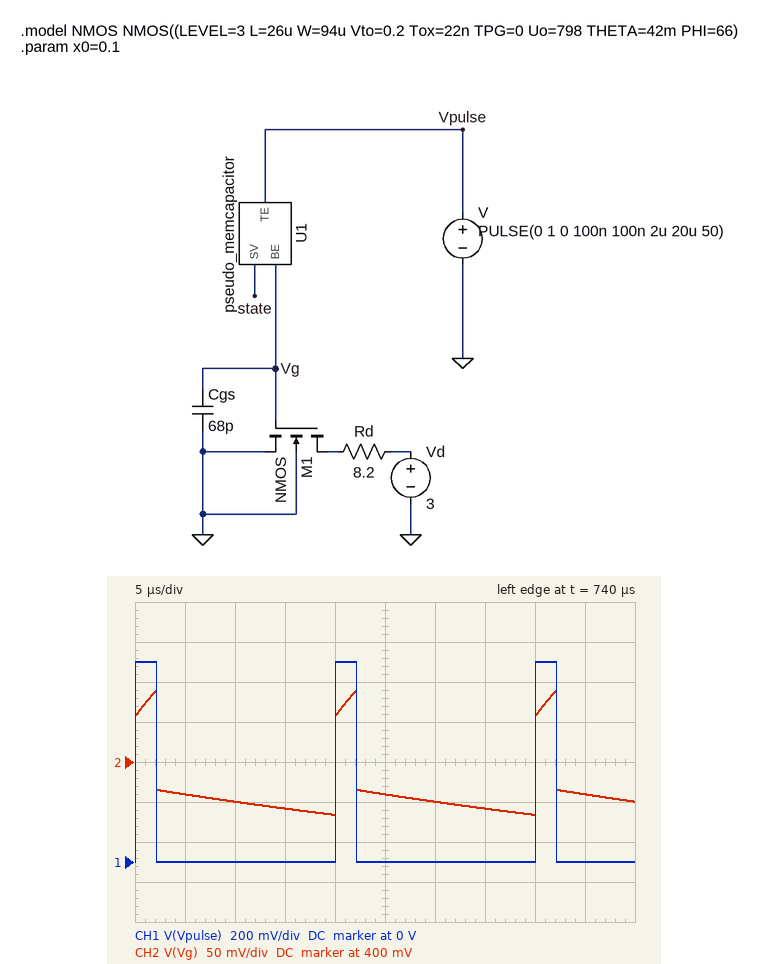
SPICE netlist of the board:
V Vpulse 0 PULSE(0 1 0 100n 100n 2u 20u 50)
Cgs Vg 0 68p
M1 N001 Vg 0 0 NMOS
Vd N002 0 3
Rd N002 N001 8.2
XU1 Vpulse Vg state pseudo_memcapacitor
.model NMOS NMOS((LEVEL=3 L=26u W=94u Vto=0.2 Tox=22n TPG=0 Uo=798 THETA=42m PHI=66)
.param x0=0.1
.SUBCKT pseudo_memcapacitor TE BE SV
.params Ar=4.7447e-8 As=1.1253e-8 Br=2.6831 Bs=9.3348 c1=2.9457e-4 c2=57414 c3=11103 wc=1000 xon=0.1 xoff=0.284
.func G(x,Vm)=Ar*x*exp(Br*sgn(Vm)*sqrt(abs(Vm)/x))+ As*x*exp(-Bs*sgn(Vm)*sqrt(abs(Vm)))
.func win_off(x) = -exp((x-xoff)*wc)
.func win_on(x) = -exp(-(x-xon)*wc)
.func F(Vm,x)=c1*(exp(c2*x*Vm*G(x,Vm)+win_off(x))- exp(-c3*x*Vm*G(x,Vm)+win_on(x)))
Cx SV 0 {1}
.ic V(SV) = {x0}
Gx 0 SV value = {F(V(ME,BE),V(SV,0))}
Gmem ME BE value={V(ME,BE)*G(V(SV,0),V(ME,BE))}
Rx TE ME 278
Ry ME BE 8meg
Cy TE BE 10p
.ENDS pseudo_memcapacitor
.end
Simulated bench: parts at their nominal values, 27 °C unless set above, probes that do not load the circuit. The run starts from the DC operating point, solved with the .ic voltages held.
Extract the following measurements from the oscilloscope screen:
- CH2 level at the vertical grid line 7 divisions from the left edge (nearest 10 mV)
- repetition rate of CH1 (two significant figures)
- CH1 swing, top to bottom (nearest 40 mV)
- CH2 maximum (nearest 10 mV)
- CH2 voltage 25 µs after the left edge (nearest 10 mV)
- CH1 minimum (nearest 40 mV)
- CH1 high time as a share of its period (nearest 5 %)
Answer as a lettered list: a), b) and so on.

a) 340 mV
b) 50 kHz
c) 1.00 V
d) 490 mV
e) 360 mV
f) 0 V
g) 10 %
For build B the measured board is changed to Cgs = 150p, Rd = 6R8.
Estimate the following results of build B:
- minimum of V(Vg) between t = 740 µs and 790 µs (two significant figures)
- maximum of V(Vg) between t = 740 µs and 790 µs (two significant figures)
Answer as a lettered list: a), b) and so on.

a) 370 mV
b) 450 mV
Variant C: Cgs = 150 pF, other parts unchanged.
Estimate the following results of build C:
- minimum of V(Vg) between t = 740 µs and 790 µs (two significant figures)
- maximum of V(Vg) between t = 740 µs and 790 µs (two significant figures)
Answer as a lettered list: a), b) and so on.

a) 370 mV
b) 450 mV
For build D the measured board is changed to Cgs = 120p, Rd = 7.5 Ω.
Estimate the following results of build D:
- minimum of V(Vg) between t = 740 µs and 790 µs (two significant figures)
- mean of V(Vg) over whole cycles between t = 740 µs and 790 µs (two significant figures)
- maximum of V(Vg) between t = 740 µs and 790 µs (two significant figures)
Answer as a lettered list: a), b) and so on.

a) 360 mV
b) 380 mV
c) 460 mV
